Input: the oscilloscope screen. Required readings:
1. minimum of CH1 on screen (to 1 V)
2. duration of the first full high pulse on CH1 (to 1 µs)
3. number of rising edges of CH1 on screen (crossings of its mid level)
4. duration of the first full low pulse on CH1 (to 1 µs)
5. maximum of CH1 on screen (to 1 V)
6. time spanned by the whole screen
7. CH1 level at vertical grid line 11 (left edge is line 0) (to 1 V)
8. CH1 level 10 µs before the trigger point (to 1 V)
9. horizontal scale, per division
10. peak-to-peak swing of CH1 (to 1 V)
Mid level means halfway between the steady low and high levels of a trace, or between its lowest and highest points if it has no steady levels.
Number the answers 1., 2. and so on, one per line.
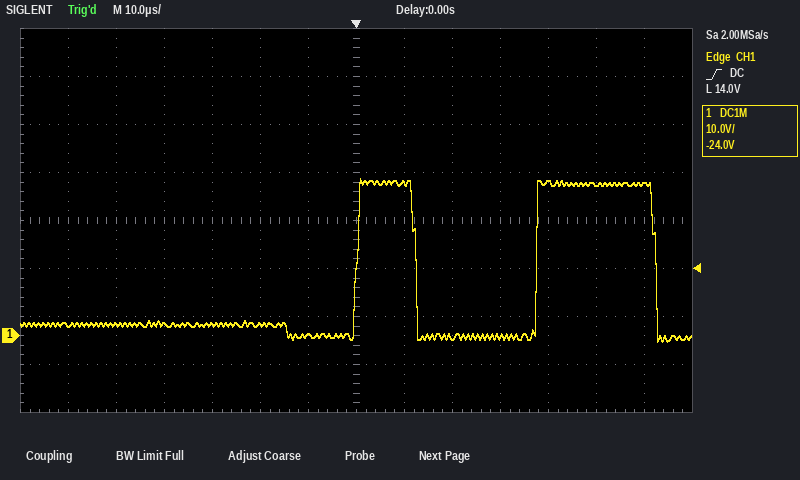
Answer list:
1. -1 V
2. 12 µs
3. 2
4. 25 µs
5. 33 V
6. 140 µs
7. 32 V
8. 0 V
9. 10 µs
10. 34 V
